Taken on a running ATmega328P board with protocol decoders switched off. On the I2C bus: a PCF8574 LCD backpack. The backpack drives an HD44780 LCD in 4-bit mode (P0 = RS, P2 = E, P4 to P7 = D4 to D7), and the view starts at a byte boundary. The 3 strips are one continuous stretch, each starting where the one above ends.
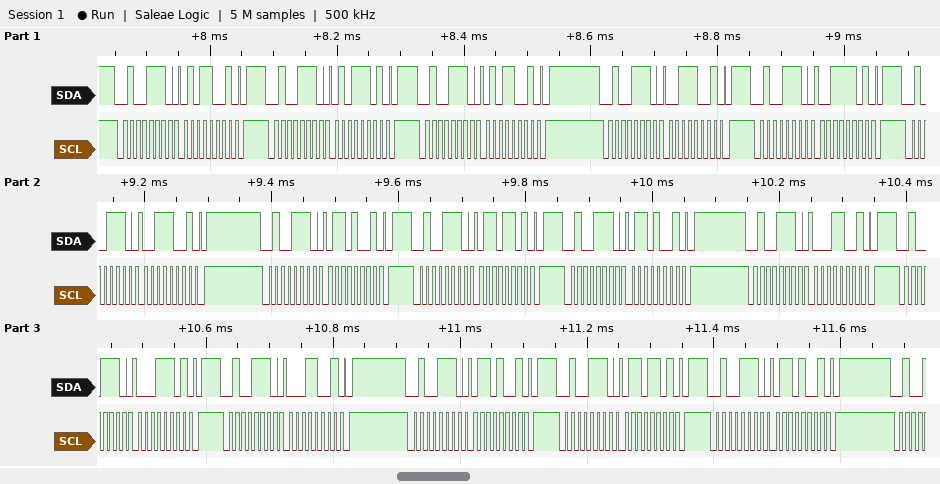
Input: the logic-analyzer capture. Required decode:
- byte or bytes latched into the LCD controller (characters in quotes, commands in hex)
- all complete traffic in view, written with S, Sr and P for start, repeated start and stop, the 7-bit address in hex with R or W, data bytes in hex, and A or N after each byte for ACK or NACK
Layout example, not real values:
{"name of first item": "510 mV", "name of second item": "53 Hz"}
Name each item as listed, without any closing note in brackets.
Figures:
{"byte or bytes latched into the LCD controller": "'S' 'a'", "all complete traffic in view, written with S, Sr and P for start, repeated start and stop, the 7-bit address in hex with R or W, data bytes in hex, and A or N after each byte for ACK or NACK": "S 27W A 59 A P S 27W A 5D A P S 27W A 59 A P S 27W A 39 A P S 27W A 3D A P S 27W A 39 A P S 27W A 69 A P S 27W A 6D A P S 27W A 69 A P S 27W A 19 A P S 27W A 1D A P S 27W A 19 A P S 27W A 69 A P S 27W A 6D A P S 27W A 69 A P"}
